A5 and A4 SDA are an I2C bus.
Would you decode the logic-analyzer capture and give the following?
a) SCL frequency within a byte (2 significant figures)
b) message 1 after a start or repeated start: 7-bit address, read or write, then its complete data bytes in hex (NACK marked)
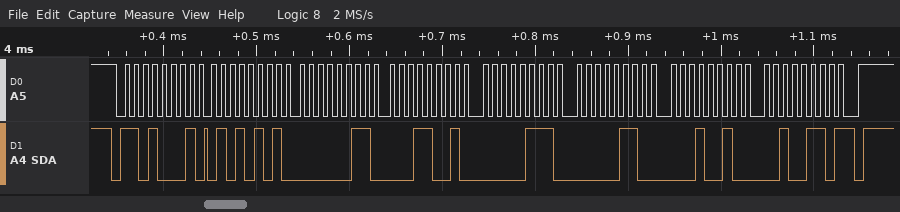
100 kHz
0x68 read: 55 03 19 07 06 12 26 NACK
